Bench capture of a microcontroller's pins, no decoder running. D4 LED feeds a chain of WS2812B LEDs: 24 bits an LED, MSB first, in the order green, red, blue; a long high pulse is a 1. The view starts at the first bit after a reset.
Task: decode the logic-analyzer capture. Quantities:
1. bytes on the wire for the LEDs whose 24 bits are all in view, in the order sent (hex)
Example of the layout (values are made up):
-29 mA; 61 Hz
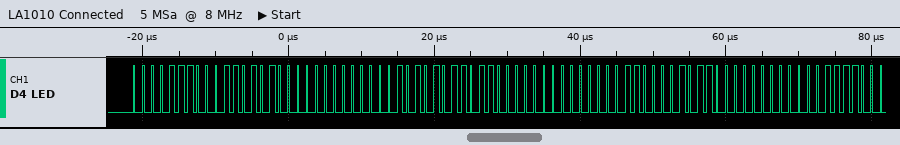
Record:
0E 35 00 05 5B 00 03 0B 00
